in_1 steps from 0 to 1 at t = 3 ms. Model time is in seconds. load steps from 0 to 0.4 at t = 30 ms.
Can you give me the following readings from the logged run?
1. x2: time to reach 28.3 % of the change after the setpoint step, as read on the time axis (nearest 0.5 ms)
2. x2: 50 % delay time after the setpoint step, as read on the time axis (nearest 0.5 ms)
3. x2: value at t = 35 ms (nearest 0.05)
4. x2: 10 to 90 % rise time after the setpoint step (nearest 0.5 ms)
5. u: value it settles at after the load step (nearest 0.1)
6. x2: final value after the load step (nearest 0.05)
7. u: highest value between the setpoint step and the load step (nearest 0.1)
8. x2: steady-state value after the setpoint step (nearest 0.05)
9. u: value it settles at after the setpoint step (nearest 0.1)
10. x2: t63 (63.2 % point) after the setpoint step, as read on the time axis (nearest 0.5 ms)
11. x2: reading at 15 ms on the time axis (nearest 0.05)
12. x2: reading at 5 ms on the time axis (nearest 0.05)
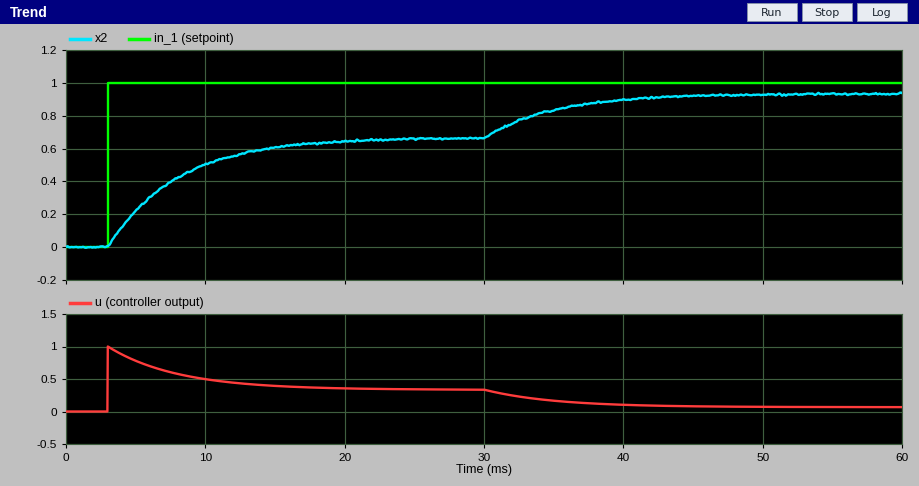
4.5 ms
6.5 ms
0.85
11.0 ms
0.1
0.95
1.0
0.65
0.3
8.0 ms
0.60
0.20
